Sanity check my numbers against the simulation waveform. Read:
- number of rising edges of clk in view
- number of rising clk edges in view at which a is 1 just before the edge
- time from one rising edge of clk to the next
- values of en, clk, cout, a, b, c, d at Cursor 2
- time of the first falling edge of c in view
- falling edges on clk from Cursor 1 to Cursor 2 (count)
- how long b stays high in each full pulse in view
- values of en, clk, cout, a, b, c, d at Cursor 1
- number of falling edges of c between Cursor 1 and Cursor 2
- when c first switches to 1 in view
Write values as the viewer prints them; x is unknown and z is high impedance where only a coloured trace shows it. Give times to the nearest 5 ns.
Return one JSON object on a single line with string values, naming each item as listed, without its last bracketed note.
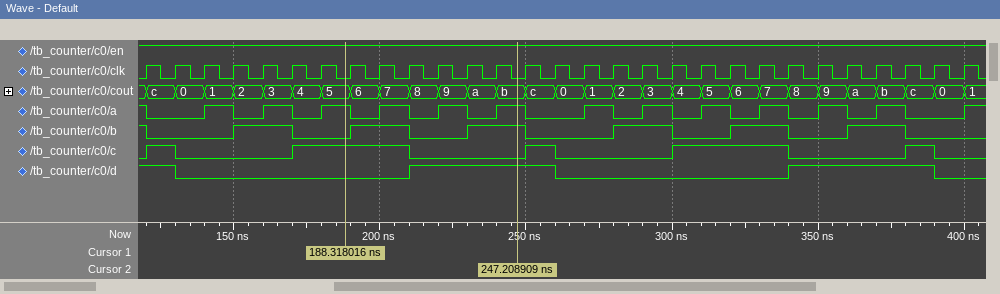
{"number of rising edges of clk in view": "29", "number of rising clk edges in view at which a is 1 just before the edge": "13", "time from one rising edge of clk to the next": "10 ns", "values of en, clk, cout, a, b, c, d at Cursor 2": "en=1, clk=0, cout=b, a=1, b=1, c=0, d=1", "time of the first falling edge of c in view": "130 ns", "falling edges on clk from Cursor 1 to Cursor 2": "6", "how long b stays high in each full pulse in view": "20 ns, 20 ns, 20 ns, 20 ns, 20 ns, 20 ns", "values of en, clk, cout, a, b, c, d at Cursor 1": "en=1, clk=0, cout=5, a=1, b=0, c=1, d=0", "number of falling edges of c between Cursor 1 and Cursor 2": "1", "when c first switches to 1 in view": "120 ns"}
